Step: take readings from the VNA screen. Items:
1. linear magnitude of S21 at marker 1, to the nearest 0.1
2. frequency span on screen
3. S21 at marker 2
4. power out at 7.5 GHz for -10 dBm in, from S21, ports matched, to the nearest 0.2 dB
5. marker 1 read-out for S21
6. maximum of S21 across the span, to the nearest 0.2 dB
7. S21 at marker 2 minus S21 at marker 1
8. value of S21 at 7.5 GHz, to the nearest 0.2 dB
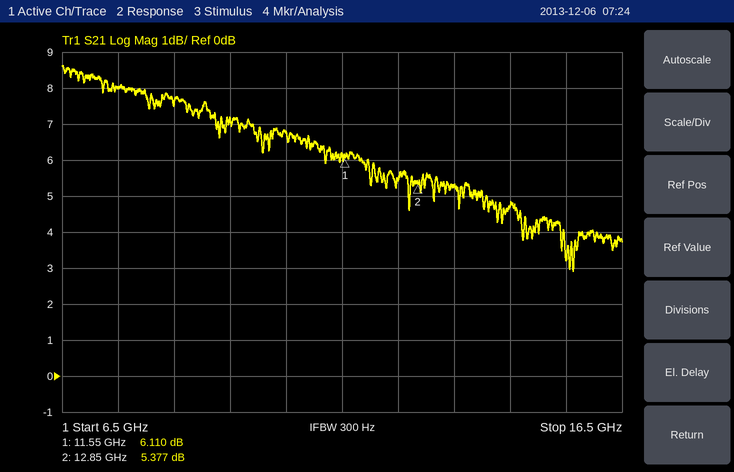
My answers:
2.0
10 GHz
5.377 dB
-2.0 dBm
6.110 dB
8.6 dB
-0.733 dB
8.0 dB
